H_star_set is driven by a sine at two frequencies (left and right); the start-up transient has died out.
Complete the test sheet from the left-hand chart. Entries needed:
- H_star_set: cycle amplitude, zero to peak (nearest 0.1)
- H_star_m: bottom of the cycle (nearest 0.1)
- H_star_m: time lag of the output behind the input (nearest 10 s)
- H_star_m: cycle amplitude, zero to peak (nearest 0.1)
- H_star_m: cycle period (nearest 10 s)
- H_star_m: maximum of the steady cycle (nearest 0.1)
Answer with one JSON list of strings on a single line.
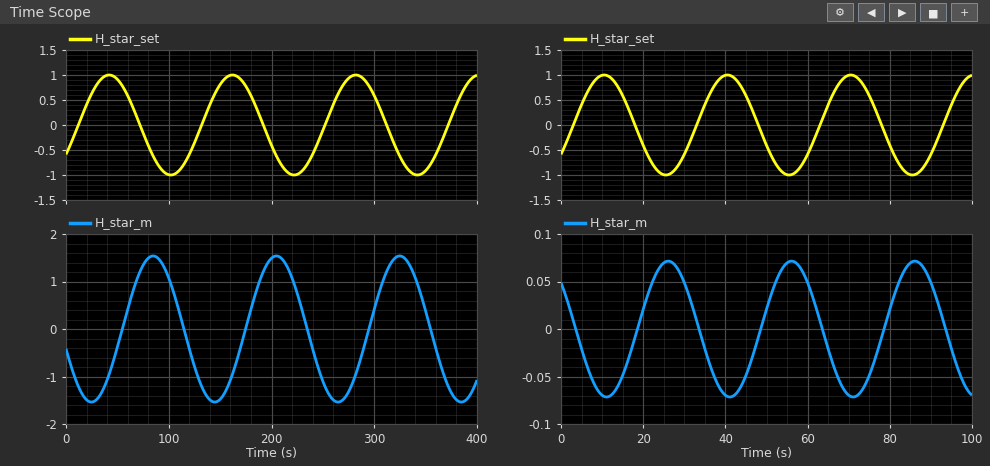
["1.0", "-1.5", "40 s", "1.5", "120 s", "1.5"]
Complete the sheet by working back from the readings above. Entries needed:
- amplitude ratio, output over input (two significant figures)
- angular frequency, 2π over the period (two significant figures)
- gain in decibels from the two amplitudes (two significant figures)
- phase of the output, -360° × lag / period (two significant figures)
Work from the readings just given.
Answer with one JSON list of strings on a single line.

["1.5", "0.052 rad/s", "3.5 dB", "-120°"]
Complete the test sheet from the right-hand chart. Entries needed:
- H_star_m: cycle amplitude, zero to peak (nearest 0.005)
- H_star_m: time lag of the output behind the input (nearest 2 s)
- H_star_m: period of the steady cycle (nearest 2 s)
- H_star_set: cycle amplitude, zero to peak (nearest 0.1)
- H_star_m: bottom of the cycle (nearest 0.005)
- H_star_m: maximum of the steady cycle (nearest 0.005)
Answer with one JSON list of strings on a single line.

["0.070", "16 s", "30 s", "1.0", "-0.070", "0.070"]
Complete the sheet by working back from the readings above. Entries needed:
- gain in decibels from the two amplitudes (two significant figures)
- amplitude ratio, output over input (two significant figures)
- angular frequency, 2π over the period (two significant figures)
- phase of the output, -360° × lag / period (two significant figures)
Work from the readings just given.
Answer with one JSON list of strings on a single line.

["-23 dB", "0.070", "0.21 rad/s", "-190°"]
